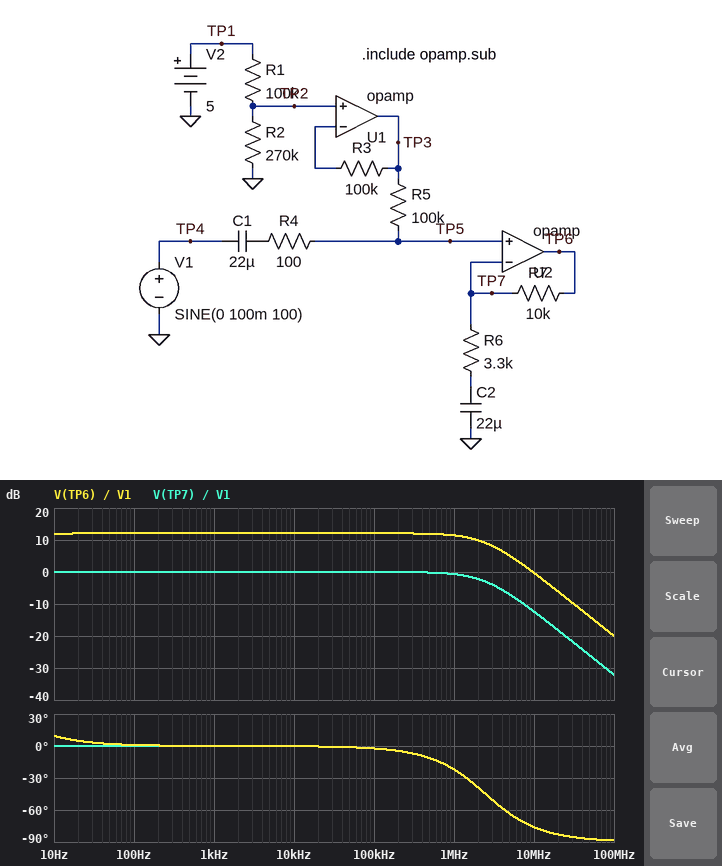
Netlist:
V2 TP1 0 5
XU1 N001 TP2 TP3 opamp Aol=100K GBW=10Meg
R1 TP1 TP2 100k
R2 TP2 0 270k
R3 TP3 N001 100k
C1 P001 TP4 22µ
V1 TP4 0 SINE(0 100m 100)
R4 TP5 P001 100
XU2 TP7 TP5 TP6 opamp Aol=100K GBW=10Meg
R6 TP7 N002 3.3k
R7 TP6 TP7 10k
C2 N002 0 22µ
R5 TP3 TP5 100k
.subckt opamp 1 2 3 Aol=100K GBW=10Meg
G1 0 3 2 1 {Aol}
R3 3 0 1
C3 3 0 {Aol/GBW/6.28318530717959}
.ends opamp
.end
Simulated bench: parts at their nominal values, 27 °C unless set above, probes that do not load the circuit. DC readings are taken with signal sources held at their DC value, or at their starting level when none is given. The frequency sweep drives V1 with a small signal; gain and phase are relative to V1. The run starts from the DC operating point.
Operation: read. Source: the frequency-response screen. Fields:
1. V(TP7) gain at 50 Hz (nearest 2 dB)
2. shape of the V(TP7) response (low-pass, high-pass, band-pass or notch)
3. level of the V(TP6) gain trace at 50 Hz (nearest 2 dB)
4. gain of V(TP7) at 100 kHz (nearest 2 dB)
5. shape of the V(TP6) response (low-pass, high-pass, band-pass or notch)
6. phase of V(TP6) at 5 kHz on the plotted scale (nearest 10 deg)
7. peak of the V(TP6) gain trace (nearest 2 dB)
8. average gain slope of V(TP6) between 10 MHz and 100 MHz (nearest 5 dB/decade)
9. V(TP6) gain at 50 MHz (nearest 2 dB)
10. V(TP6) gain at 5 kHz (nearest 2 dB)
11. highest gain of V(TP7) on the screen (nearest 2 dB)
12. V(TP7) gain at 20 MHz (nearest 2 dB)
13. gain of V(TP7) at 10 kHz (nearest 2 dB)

0 dB
low-pass
12 dB
0 dB
low-pass
0 deg
12 dB
-20 dB/decade
-14 dB
12 dB
0 dB
-18 dB
0 dB
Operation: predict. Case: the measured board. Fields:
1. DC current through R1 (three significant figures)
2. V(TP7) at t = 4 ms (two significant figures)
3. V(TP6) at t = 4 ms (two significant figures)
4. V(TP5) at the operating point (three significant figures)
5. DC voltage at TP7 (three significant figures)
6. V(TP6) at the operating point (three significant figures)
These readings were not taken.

13.5 µA
3.7 V
3.9 V
3.65 V
3.65 V
3.65 V
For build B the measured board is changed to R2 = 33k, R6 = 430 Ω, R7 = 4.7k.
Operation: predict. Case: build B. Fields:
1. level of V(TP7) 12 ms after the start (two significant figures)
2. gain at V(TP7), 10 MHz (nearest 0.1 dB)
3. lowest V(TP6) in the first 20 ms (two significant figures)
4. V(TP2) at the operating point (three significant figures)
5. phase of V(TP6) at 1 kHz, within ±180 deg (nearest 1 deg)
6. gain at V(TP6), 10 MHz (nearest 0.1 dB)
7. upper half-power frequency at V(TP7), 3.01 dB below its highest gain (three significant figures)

1.3 V
-21.6 dB
-18 mV
1.24 V
1 deg
0 dB
838 kHz
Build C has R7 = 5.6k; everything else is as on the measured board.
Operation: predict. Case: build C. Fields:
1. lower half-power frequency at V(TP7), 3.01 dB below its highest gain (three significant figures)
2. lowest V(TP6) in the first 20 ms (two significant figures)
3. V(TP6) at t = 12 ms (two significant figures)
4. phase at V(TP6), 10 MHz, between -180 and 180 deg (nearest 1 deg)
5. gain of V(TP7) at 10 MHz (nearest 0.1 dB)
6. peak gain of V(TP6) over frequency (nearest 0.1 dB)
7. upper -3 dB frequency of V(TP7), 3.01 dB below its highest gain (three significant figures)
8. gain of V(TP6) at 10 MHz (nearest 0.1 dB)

72.3 mHz
3.4 V
3.9 V
-70 deg
-9.2 dB
8.6 dB
3.71 MHz
-0.6 dB
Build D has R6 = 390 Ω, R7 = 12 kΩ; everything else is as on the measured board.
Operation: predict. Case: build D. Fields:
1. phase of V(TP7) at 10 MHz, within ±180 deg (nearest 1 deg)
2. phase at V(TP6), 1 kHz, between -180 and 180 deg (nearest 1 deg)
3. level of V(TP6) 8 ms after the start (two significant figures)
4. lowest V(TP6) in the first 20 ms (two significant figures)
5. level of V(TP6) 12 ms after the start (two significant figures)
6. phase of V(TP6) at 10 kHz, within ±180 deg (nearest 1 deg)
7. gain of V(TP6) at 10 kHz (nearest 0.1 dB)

-88 deg
1 deg
680 mV
290 mV
6.6 V
-2 deg
30.0 dB
